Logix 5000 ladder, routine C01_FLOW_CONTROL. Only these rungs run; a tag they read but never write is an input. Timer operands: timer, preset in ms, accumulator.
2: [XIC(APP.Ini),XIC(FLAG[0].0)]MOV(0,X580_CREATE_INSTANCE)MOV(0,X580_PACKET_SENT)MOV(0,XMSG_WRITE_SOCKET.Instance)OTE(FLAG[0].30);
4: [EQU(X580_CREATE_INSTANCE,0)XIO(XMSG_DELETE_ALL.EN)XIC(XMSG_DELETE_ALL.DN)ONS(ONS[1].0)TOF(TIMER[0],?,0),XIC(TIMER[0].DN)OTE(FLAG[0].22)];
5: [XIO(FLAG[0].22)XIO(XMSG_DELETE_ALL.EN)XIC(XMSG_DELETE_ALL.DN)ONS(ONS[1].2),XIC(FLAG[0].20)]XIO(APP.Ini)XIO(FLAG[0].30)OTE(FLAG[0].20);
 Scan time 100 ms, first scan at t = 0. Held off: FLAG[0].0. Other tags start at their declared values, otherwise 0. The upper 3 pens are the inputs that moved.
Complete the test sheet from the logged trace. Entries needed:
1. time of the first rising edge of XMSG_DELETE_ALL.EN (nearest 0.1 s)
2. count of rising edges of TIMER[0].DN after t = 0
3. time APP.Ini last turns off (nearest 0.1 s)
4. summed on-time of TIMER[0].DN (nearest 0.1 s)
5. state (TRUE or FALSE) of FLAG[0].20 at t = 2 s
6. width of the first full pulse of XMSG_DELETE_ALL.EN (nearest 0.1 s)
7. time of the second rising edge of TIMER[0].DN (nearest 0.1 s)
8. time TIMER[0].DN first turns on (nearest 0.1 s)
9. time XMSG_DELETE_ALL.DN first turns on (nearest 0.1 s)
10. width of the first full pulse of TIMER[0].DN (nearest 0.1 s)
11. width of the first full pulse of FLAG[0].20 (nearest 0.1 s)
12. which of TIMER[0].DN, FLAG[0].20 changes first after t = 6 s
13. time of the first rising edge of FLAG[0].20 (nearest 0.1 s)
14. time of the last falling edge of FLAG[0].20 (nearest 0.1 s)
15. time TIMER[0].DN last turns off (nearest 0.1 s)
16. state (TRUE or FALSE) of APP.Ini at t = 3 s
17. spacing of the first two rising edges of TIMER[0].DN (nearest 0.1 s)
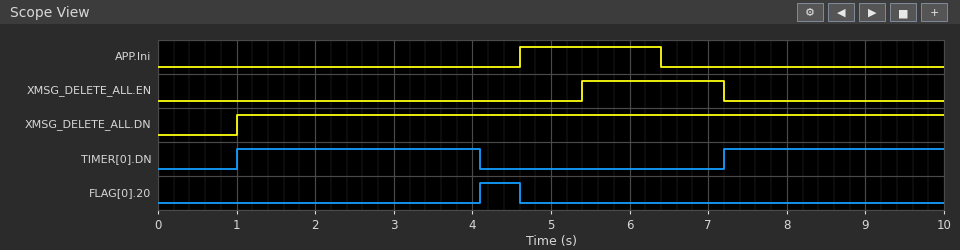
5.4 s
2
6.4 s
5.9 s
FALSE
1.8 s
7.2 s
1.0 s
1.0 s
3.1 s
0.5 s
TIMER[0].DN
4.1 s
4.6 s
4.1 s
FALSE
6.2 s
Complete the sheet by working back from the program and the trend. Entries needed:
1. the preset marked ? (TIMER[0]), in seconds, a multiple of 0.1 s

3.0 s
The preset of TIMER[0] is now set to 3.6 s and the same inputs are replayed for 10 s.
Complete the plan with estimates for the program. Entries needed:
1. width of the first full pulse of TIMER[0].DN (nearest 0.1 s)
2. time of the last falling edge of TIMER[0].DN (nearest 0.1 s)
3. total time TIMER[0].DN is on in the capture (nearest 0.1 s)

3.7 s
4.7 s
6.5 s
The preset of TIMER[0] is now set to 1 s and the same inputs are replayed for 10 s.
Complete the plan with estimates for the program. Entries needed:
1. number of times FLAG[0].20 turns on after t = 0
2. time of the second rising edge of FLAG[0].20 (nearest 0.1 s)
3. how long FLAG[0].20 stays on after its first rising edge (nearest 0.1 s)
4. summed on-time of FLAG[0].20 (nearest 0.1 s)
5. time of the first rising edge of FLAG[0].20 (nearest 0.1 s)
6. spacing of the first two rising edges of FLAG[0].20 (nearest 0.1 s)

2
8.3 s
2.5 s
4.2 s
2.1 s
6.2 s
